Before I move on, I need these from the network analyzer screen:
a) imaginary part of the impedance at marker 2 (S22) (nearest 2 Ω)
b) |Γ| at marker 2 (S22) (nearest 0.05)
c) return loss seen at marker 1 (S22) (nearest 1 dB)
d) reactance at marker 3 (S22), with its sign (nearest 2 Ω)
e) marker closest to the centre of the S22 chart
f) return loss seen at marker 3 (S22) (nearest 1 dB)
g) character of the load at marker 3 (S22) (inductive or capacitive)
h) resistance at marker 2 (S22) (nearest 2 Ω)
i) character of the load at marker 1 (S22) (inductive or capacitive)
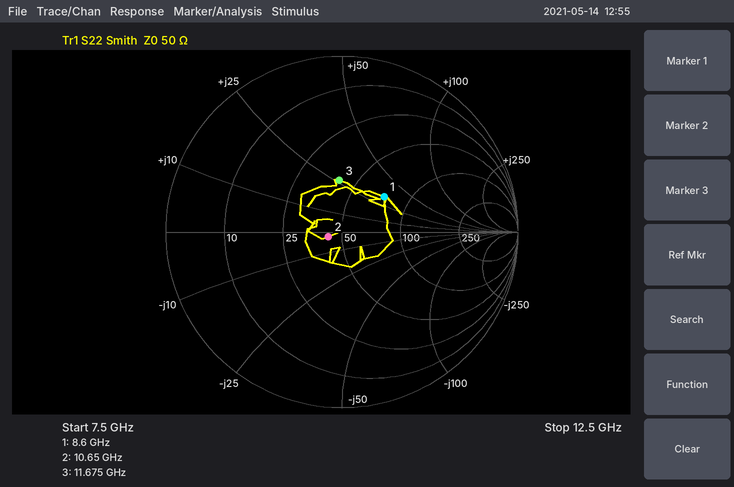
-2 Ω
0.10
10 dB
+26 Ω
marker 2
11 dB
inductive
42 Ω
inductive
